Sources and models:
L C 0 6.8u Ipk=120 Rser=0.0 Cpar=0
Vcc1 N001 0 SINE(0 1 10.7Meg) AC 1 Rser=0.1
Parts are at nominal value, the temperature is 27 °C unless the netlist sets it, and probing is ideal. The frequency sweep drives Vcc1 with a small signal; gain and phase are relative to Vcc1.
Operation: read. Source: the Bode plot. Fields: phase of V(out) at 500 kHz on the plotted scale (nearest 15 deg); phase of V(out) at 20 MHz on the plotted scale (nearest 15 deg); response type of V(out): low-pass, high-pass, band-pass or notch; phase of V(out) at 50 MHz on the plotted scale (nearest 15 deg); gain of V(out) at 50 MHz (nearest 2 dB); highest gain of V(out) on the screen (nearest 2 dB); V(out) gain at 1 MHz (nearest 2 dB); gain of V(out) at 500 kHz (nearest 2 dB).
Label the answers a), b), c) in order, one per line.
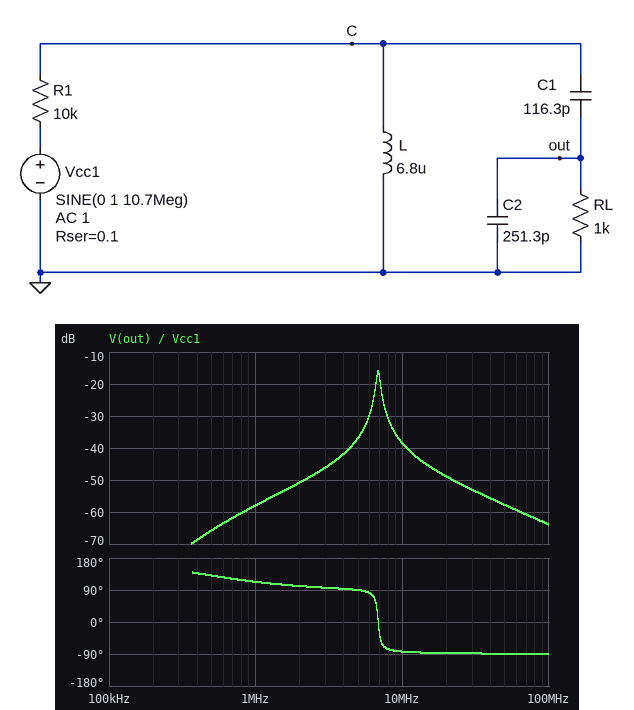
a) 135 deg
b) -90 deg
c) band-pass
d) -90 deg
e) -58 dB
f) -16 dB
g) -58 dB
h) -66 dB
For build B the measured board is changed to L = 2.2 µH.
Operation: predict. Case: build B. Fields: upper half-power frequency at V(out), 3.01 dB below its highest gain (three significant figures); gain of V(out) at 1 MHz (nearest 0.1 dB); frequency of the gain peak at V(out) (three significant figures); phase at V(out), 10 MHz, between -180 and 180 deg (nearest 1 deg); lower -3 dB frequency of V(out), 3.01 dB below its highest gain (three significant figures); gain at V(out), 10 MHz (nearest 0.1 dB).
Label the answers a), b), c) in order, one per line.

a) 12.2 MHz
b) -67.9 dB
c) 12.0 MHz
d) 87 deg
e) 11.8 MHz
f) -37.0 dB
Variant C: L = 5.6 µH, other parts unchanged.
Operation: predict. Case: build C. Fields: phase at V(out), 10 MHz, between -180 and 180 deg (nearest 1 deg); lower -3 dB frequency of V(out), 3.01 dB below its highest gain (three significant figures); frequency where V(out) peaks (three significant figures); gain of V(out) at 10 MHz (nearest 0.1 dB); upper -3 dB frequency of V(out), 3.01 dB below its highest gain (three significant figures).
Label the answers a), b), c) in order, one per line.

a) -82 deg
b) 7.34 MHz
c) 7.54 MHz
d) -36.7 dB
e) 7.74 MHz
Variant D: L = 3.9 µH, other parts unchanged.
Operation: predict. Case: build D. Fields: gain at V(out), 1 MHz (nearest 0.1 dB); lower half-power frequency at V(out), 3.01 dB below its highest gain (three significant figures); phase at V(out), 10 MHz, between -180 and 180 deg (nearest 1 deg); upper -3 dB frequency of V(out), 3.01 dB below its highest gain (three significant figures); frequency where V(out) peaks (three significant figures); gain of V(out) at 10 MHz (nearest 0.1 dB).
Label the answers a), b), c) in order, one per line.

a) -62.8 dB
b) 8.84 MHz
c) -75 deg
d) 9.24 MHz
e) 9.03 MHz
f) -29.5 dB
